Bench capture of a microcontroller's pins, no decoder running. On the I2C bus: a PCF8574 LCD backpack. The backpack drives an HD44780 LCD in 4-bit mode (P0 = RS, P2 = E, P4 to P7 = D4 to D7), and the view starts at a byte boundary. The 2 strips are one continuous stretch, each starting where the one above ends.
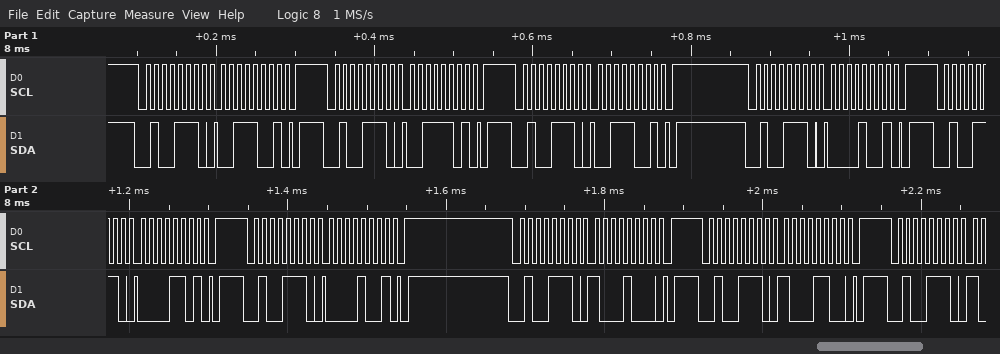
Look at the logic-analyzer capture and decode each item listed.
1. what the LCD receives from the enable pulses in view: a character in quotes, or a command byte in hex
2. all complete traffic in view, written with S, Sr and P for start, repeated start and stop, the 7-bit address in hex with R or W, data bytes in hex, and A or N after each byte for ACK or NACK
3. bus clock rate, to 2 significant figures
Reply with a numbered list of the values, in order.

1. '0'
2. S 27W A 39 A P S 27W A 3D A P S 27W A 39 A P S 27W A 09 A P S 27W A 0D A P S 27W A 09 A P S 27W A 88 A P S 27W A 8C A P S 27W A
3. 100 kHz
